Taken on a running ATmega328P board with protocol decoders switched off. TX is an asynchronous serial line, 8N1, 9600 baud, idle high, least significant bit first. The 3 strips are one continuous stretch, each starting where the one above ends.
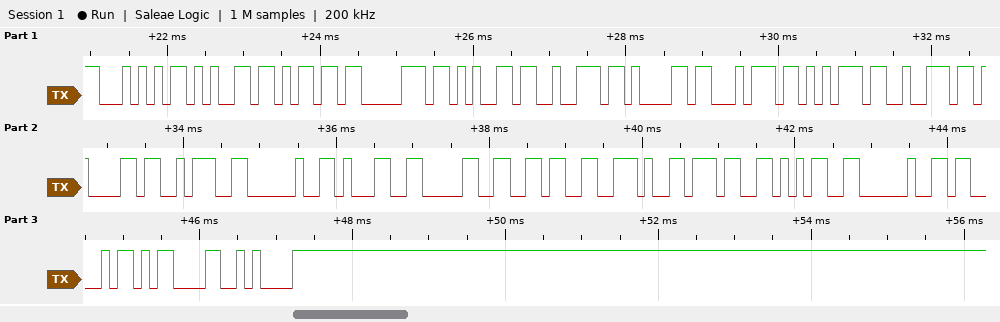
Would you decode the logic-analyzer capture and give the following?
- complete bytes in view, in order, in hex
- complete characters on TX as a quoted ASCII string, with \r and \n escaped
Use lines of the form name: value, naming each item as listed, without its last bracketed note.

complete bytes in view, in order, in hex: 0x54 0x65 0x6D 0x70 0x65 0x72 0x61 0x74 0x75 0x72 0x61 0x3A 0x20 0x31 0x30 0x36 0x2E 0x37 0x35 0x20 0x43 0x0D 0x0A
complete characters on TX as a quoted ASCII string, with \r and \n escaped: "Temperatura: 106.75 C\r\n"
